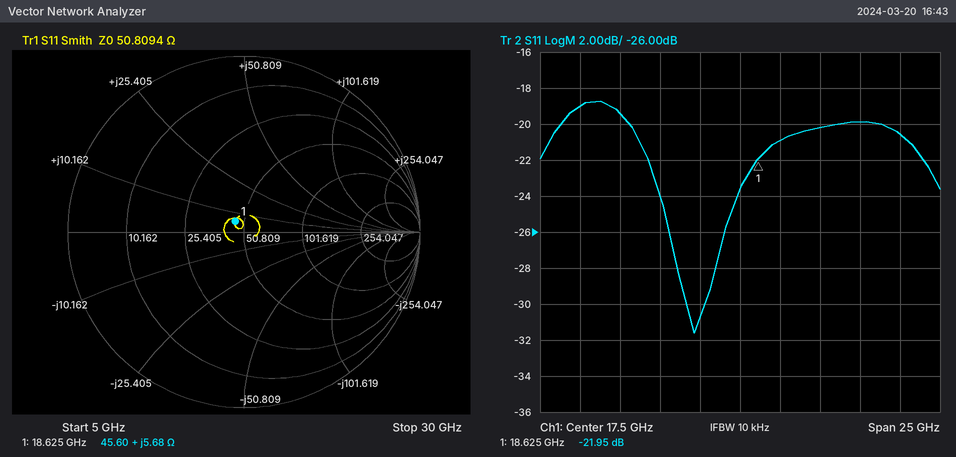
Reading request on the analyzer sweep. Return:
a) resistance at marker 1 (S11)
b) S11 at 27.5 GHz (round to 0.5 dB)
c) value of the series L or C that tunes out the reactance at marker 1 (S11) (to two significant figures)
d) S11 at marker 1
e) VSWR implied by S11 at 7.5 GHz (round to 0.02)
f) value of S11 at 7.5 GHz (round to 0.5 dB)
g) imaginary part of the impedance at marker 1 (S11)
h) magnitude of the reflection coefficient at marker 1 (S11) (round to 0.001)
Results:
45.60 Ω
-20.5 dB
1.5 pF
-21.95 dB
1.26
-19.0 dB
+5.68 Ω
0.080
